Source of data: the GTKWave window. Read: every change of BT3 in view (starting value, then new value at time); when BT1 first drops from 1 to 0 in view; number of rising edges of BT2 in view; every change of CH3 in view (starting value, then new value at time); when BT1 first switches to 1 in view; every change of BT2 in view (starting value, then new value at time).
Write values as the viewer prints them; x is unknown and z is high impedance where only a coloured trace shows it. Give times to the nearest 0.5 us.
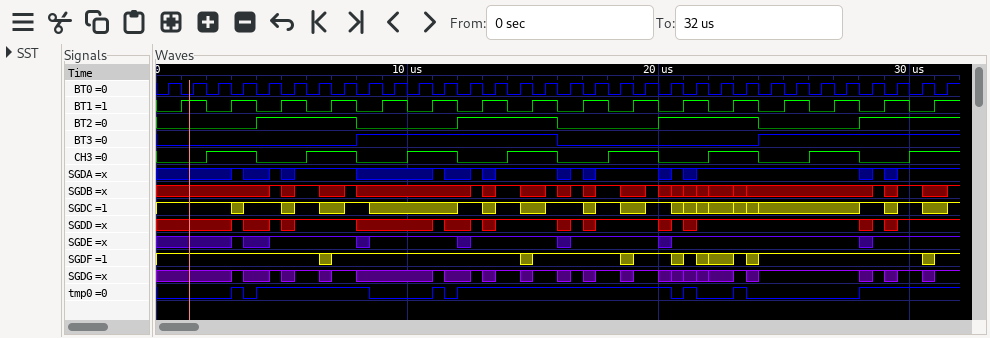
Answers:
0, 1 at 8 us, 0 at 16 us, 1 at 24 us
2 us
4
0, 1 at 2 us, 0 at 4 us, 1 at 6 us, 0 at 8 us, 1 at 10 us, 0 at 12 us, 1 at 14 us, 0 at 16 us, 1 at 18 us, 0 at 20 us, 1 at 22 us, 0 at 24 us, 1 at 26 us, 0 at 28 us, 1 at 30 us
1 us
0, 1 at 4 us, 0 at 8 us, 1 at 12 us, 0 at 16 us, 1 at 20 us, 0 at 24 us, 1 at 28 us
